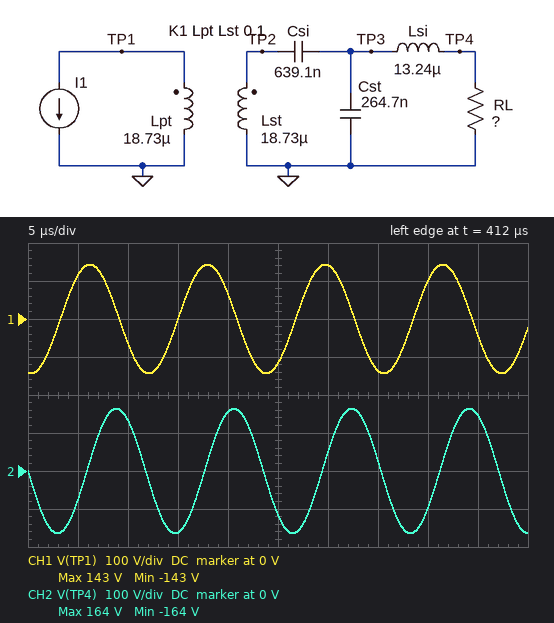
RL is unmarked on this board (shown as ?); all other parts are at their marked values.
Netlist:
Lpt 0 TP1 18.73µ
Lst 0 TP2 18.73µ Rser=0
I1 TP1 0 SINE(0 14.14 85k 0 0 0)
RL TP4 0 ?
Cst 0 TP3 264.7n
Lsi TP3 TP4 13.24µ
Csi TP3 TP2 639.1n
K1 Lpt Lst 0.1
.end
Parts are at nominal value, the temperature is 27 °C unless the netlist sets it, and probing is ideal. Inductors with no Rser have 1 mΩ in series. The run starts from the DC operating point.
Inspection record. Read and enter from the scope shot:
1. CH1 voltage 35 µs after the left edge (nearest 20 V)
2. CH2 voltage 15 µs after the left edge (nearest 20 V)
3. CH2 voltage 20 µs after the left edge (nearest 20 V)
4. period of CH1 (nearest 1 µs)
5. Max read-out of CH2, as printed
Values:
-140 V
-160 V
160 V
12 µs
164 V
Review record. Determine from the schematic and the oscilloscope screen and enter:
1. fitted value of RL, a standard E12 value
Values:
82 Ω
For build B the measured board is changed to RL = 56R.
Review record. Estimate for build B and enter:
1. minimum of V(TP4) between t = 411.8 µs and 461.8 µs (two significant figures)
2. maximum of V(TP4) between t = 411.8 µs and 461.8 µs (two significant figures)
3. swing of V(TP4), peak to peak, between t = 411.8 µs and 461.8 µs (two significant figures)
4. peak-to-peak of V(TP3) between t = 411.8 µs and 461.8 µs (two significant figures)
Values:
-110 V
110 V
220 V
230 V
